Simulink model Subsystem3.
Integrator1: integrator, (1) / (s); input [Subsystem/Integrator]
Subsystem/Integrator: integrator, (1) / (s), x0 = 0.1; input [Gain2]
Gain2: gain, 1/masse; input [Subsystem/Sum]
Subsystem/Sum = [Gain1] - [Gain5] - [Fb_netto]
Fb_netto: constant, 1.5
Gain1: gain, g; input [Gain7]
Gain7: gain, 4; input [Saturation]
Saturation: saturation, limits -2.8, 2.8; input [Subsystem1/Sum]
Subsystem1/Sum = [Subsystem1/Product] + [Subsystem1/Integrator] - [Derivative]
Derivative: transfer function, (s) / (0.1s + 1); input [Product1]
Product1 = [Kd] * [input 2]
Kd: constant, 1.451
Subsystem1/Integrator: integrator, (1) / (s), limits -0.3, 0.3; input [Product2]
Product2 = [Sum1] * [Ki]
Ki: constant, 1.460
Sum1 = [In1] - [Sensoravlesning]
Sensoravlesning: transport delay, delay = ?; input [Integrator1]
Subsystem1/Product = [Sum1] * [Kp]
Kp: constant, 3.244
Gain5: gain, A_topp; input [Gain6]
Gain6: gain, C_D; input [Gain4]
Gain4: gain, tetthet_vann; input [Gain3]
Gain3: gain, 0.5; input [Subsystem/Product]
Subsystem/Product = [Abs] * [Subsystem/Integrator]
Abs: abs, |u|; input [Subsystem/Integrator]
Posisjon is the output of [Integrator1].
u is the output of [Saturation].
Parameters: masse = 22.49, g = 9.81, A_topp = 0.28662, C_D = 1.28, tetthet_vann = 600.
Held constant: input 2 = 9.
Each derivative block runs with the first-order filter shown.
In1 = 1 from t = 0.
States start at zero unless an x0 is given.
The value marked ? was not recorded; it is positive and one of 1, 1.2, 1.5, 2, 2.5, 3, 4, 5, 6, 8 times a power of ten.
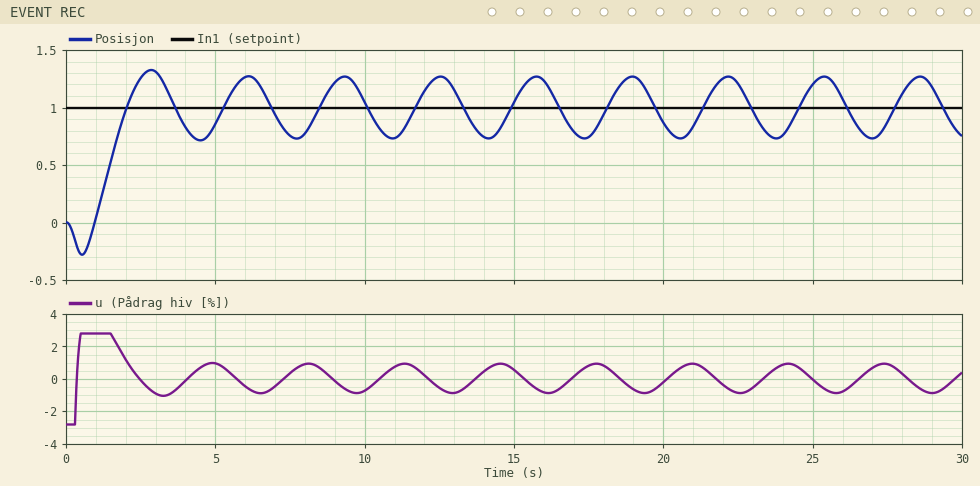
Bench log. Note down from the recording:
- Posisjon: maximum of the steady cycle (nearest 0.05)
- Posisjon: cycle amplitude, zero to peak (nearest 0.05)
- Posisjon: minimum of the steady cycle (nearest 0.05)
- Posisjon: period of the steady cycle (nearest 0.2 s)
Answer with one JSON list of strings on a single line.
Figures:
["1.25", "0.25", "0.75", "3.2 s"]
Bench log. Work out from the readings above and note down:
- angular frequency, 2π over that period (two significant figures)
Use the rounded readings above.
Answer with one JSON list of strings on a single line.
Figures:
["2.0 rad/s"]
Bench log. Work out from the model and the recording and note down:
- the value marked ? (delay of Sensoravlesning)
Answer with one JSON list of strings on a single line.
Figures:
["0.3"]
